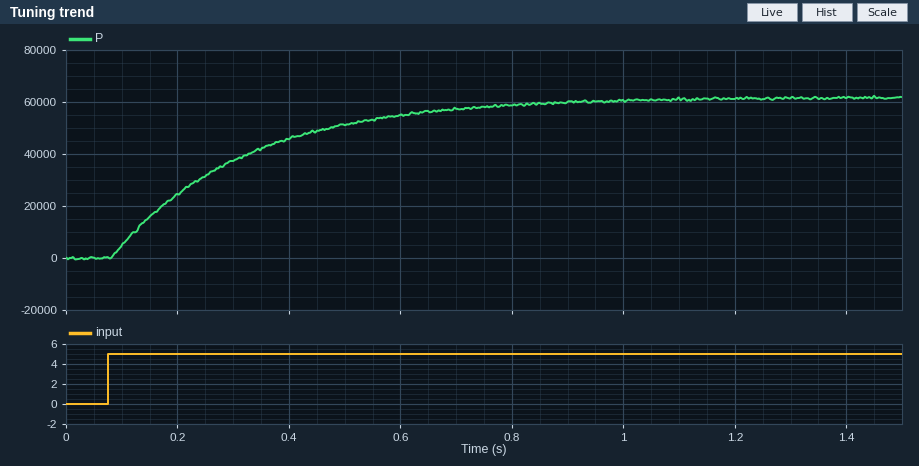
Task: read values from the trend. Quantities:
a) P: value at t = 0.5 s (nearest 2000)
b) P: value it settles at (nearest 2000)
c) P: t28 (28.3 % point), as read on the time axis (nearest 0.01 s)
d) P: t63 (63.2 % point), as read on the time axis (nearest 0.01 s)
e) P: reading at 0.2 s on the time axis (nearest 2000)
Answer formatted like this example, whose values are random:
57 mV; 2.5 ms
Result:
52000; 62000; 0.16 s; 0.32 s; 24000
